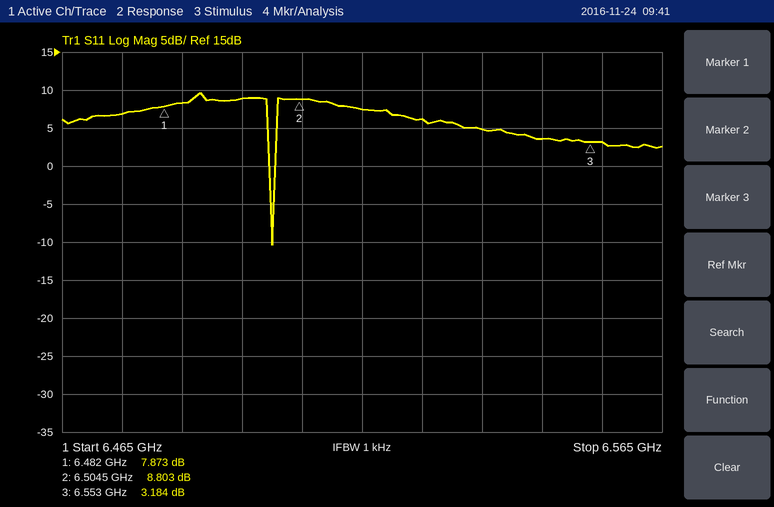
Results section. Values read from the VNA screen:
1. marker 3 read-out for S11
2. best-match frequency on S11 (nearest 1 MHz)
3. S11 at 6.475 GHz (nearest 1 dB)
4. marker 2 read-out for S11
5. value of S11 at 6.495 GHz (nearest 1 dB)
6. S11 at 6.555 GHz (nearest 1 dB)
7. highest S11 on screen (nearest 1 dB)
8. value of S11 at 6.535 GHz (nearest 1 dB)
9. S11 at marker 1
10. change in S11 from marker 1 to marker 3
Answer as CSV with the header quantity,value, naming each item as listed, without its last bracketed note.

quantity,value
marker 3 read-out for S11,3.184 dB
best-match frequency on S11,6.500 GHz
S11 at 6.475 GHz,7 dB
marker 2 read-out for S11,8.803 dB
value of S11 at 6.495 GHz,9 dB
S11 at 6.555 GHz,3 dB
highest S11 on screen,10 dB
value of S11 at 6.535 GHz,5 dB
S11 at marker 1,7.873 dB
change in S11 from marker 1 to marker 3,-4.689 dB
